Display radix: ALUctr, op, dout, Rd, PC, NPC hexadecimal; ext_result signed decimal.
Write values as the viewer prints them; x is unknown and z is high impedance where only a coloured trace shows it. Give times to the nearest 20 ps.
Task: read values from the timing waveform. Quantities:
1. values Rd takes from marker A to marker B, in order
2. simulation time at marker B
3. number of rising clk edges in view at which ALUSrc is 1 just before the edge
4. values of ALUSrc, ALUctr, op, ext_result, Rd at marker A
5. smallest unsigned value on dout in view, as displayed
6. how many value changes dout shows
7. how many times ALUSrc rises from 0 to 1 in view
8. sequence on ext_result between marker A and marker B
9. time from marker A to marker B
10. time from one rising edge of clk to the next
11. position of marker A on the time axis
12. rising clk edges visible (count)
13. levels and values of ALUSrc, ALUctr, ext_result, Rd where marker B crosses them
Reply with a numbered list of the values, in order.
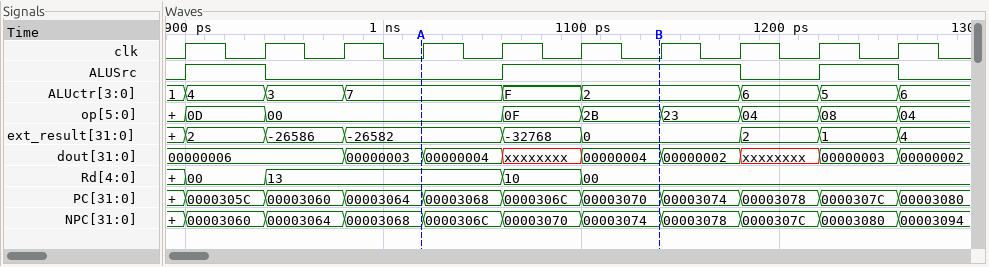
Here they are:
1. 13, 10, 00
2. 1140 ps
3. 5
4. ALUSrc=0, ALUctr=7, op=00, ext_result=-26582, Rd=13
5. 00000002
6. 8
7. 3
8. -26582, -32768, 0
9. 120 ps
10. 40 ps
11. 1020 ps
12. 10
13. ALUSrc=1, ALUctr=2, ext_result=0, Rd=00
